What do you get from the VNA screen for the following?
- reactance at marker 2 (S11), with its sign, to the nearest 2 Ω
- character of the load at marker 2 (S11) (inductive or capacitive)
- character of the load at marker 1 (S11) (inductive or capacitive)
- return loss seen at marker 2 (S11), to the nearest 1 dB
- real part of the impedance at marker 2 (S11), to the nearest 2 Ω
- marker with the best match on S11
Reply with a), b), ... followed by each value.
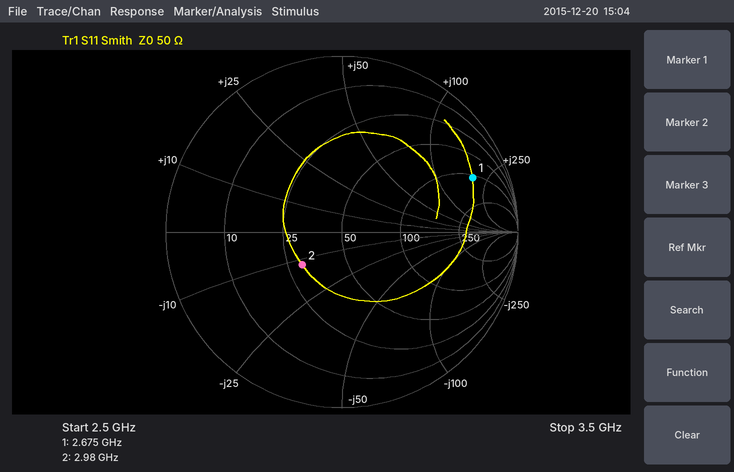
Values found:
a) -12 Ω
b) capacitive
c) inductive
d) 11 dB
e) 30 Ω
f) marker 2
